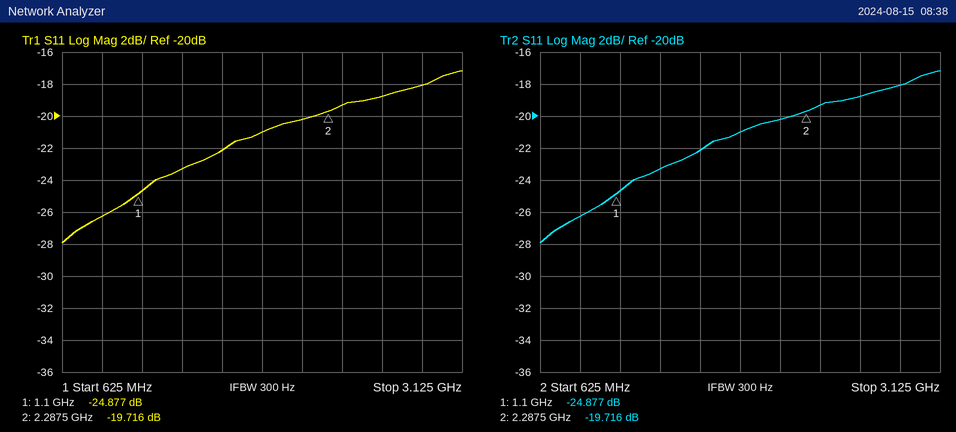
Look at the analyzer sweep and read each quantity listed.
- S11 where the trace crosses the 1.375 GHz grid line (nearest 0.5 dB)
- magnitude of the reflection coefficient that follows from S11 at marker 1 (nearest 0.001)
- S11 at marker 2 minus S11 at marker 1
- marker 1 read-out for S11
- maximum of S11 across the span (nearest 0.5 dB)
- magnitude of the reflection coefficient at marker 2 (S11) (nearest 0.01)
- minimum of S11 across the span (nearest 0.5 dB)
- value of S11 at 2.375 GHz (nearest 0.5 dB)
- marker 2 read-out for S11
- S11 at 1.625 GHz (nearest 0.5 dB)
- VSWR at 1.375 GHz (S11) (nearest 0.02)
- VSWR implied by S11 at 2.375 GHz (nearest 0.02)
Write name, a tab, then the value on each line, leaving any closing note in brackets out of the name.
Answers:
S11 where the trace crosses the 1.375 GHz grid line	-23.5 dB
magnitude of the reflection coefficient that follows from S11 at marker 1	0.057
S11 at marker 2 minus S11 at marker 1	5.161 dB
marker 1 read-out for S11	-24.877 dB
maximum of S11 across the span	-17.0 dB
magnitude of the reflection coefficient at marker 2 (S11)	0.10
minimum of S11 across the span	-28.0 dB
value of S11 at 2.375 GHz	-19.5 dB
marker 2 read-out for S11	-19.716 dB
S11 at 1.625 GHz	-22.0 dB
VSWR at 1.375 GHz (S11)	1.14
VSWR implied by S11 at 2.375 GHz	1.24
